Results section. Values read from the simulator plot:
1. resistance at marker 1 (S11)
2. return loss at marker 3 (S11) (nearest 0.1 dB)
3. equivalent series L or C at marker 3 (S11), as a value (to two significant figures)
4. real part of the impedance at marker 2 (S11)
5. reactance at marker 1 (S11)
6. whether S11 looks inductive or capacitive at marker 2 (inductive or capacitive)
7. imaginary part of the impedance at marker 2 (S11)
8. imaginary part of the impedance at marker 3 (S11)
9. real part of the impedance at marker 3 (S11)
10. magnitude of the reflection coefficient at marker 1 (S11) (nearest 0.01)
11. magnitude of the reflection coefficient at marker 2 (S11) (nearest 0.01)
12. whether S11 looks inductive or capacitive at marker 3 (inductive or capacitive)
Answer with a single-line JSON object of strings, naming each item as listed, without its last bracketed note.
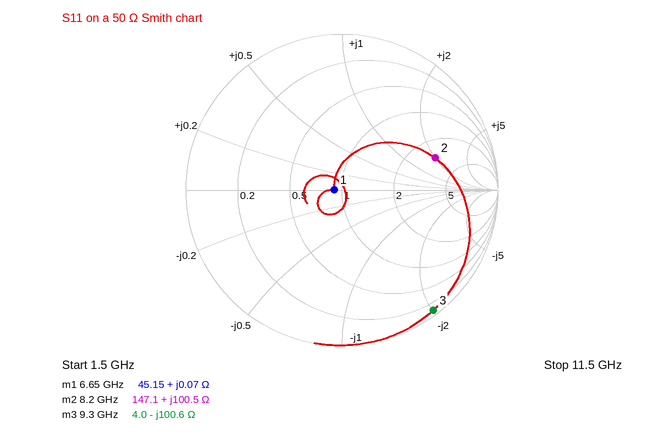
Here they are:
{"resistance at marker 1": "45.15 Ω", "return loss at marker 3 (S11)": "0.3 dB", "equivalent series L or C at marker 3 (S11), as a value": "170 fF", "real part of the impedance at marker 2": "147.1 Ω", "reactance at marker 1": "+0.07 Ω", "whether S11 looks inductive or capacitive at marker 2": "inductive", "imaginary part of the impedance at marker 2": "+100.5 Ω", "imaginary part of the impedance at marker 3": "-100.6 Ω", "real part of the impedance at marker 3": "4.0 Ω", "magnitude of the reflection coefficient at marker 1 (S11)": "0.05", "magnitude of the reflection coefficient at marker 2 (S11)": "0.63", "whether S11 looks inductive or capacitive at marker 3": "capacitive"}
